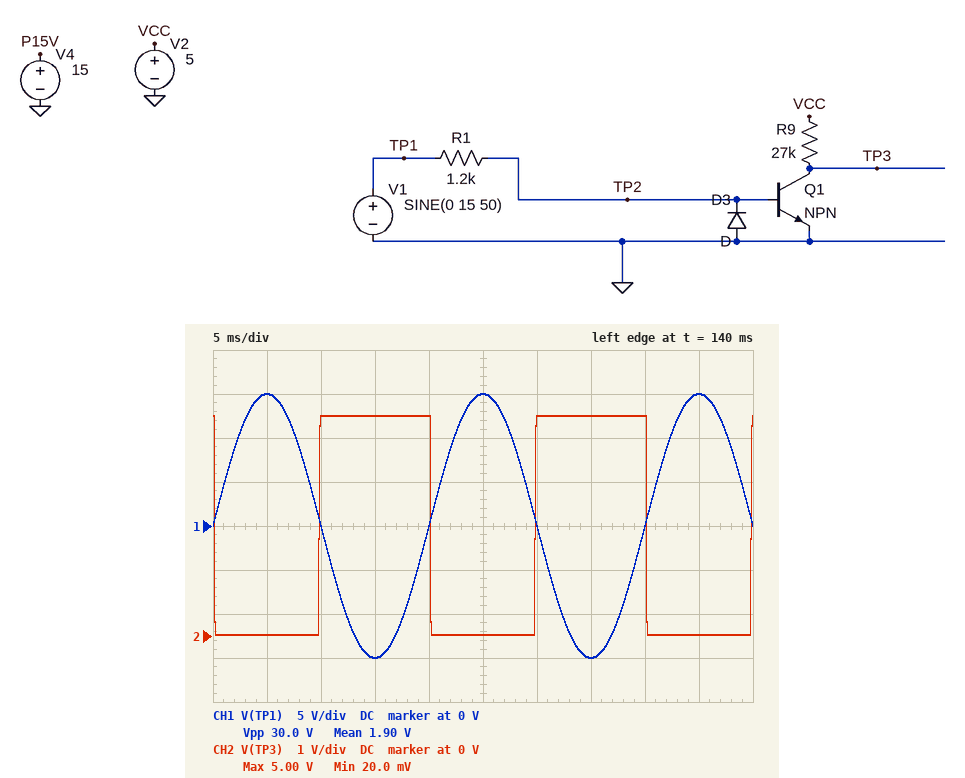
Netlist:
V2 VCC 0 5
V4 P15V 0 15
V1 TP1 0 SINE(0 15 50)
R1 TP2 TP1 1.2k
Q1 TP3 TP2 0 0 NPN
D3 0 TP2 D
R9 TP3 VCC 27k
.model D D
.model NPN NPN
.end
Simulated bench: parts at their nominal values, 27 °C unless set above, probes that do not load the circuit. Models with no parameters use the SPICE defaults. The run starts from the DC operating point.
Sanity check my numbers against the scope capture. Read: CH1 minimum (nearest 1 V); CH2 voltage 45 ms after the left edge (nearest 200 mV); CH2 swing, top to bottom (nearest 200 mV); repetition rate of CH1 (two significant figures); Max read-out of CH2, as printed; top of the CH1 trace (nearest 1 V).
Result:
-15 V
0 V
5.0 V
50 Hz
5.00 V
15 V
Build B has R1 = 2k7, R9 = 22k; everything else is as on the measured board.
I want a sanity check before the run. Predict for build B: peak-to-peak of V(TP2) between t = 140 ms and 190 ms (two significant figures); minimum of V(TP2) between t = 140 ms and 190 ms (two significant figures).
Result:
1.5 V
-700 mV
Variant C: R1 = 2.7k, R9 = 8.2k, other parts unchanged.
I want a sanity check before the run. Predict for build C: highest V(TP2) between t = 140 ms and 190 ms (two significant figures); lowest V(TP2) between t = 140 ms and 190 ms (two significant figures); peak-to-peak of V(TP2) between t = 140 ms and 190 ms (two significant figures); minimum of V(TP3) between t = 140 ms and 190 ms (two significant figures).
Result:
840 mV
-700 mV
1.5 V
19 mV
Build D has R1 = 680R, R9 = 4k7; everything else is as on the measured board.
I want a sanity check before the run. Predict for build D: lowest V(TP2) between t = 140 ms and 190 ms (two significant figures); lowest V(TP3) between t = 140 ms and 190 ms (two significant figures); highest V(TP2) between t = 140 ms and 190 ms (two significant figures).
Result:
-730 mV
19 mV
870 mV
